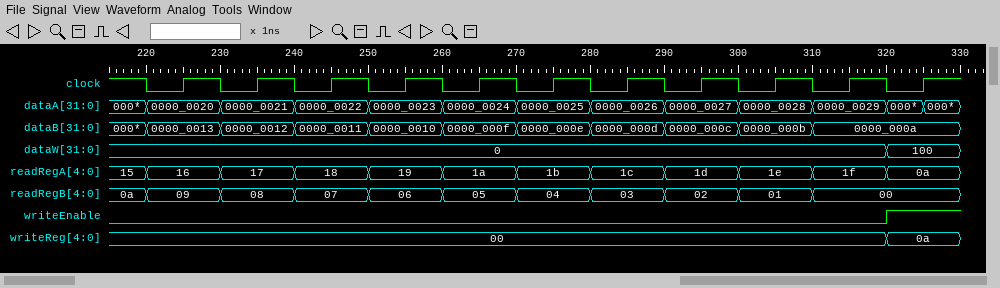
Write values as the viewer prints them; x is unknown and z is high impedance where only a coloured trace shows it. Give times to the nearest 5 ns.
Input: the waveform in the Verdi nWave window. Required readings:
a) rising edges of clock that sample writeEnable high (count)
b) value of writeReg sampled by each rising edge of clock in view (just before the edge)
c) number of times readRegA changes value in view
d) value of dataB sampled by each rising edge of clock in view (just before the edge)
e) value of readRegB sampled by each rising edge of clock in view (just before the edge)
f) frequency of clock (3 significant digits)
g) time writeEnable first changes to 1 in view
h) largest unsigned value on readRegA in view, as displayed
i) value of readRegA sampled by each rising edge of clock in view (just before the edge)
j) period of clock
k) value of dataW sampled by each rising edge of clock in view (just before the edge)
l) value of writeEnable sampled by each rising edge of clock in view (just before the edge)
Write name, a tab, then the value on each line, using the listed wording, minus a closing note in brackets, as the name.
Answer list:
rising edges of clock that sample writeEnable high	1
value of writeReg sampled by each rising edge of clock in view	00, 00, 00, 00, 00, 00, 00, 00, 00, 00, 0a
number of times readRegA changes value in view	11
value of dataB sampled by each rising edge of clock in view	0000_0013, 0000_0012, 0000_0011, 0000_0010, 0000_000f, 0000_000e, 0000_000d, 0000_000c, 0000_000b, 0000_000a, 0000_000a
value of readRegB sampled by each rising edge of clock in view	09, 08, 07, 06, 05, 04, 03, 02, 01, 00, 00
frequency of clock	100 MHz
time writeEnable first changes to 1 in view	320 ns
largest unsigned value on readRegA in view, as displayed	1f
value of readRegA sampled by each rising edge of clock in view	16, 17, 18, 19, 1a, 1b, 1c, 1d, 1e, 1f, 0a
period of clock	10 ns
value of dataW sampled by each rising edge of clock in view	0, 0, 0, 0, 0, 0, 0, 0, 0, 0, 100
value of writeEnable sampled by each rising edge of clock in view	0 0 0 0 0 0 0 0 0 0 1
